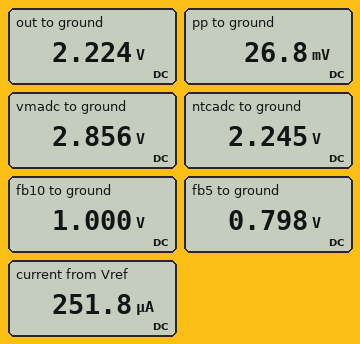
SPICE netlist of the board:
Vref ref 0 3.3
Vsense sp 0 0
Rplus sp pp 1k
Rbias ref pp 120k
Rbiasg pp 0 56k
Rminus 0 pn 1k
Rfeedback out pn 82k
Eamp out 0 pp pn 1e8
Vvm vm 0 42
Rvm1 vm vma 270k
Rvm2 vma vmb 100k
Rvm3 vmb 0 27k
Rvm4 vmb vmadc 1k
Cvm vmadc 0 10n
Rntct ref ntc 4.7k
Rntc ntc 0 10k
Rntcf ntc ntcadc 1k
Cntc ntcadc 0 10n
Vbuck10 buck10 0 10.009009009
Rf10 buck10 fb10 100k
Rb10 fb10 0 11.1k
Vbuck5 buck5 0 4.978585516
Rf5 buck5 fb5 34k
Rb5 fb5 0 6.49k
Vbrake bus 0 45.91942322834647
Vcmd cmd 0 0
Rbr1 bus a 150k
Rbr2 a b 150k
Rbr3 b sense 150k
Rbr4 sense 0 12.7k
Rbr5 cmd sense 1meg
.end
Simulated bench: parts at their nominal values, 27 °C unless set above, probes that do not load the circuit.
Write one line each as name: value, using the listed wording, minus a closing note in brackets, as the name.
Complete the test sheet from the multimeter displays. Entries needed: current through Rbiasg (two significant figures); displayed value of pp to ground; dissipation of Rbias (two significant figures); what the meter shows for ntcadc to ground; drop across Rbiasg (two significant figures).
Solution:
current through Rbiasg: 480 nA
displayed value of pp to ground: 26.8 mV
dissipation of Rbias: 89 µW
what the meter shows for ntcadc to ground: 2.245 V
drop across Rbiasg: 27 mV
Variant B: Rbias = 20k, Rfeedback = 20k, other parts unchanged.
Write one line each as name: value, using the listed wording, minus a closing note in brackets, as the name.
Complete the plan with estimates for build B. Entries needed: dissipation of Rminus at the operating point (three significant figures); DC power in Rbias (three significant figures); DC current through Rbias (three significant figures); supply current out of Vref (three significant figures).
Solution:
dissipation of Rminus at the operating point: 23.9 µW
DC power in Rbias: 495 µW
DC current through Rbias: 157 µA
supply current out of Vref: 382 µA
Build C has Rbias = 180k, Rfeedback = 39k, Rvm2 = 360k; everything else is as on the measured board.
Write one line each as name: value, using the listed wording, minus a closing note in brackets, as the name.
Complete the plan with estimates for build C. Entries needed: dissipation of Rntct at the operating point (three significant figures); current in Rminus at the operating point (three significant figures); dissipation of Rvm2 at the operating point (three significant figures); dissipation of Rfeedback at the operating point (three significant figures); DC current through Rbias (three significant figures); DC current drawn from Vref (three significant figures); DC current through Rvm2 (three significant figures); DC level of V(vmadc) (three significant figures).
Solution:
dissipation of Rntct at the operating point: 237 µW
current in Rminus at the operating point: 17.9 µA
dissipation of Rvm2 at the operating point: 1.47 mW
dissipation of Rfeedback at the operating point: 12.5 µW
DC current through Rbias: 18.2 µA
DC current drawn from Vref: 243 µA
DC current through Rvm2: 63.9 µA
DC level of V(vmadc): 1.73 V
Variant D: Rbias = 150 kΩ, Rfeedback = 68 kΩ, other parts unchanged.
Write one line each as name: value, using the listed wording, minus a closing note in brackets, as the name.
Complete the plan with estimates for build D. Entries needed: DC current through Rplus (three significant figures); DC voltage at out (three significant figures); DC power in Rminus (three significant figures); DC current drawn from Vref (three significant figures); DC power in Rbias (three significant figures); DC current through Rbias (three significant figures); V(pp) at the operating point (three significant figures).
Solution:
DC current through Rplus: 21.5 µA
DC voltage at out: 1.48 V
DC power in Rminus: 461 nW
DC current drawn from Vref: 246 µA
DC power in Rbias: 71.7 µW
DC current through Rbias: 21.9 µA
V(pp) at the operating point: 21.5 mV
